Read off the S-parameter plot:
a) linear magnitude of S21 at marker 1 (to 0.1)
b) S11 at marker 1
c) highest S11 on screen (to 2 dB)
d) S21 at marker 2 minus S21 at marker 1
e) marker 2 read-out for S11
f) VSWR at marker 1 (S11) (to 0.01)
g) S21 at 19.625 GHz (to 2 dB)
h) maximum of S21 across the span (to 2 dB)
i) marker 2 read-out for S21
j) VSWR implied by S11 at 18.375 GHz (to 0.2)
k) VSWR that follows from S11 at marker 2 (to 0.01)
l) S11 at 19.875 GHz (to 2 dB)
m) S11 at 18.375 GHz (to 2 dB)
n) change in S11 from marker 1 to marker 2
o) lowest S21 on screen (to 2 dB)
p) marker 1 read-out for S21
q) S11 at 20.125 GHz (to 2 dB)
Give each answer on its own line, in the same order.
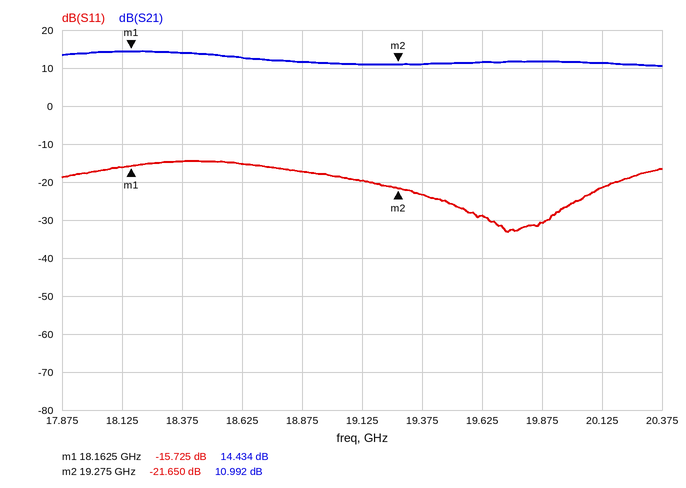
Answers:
5.3
-15.725 dB
-14 dB
-3.442 dB
-21.650 dB
1.39
12 dB
14 dB
10.992 dB
1.4
1.18
-30 dB
-14 dB
-5.925 dB
10 dB
14.434 dB
-22 dB
